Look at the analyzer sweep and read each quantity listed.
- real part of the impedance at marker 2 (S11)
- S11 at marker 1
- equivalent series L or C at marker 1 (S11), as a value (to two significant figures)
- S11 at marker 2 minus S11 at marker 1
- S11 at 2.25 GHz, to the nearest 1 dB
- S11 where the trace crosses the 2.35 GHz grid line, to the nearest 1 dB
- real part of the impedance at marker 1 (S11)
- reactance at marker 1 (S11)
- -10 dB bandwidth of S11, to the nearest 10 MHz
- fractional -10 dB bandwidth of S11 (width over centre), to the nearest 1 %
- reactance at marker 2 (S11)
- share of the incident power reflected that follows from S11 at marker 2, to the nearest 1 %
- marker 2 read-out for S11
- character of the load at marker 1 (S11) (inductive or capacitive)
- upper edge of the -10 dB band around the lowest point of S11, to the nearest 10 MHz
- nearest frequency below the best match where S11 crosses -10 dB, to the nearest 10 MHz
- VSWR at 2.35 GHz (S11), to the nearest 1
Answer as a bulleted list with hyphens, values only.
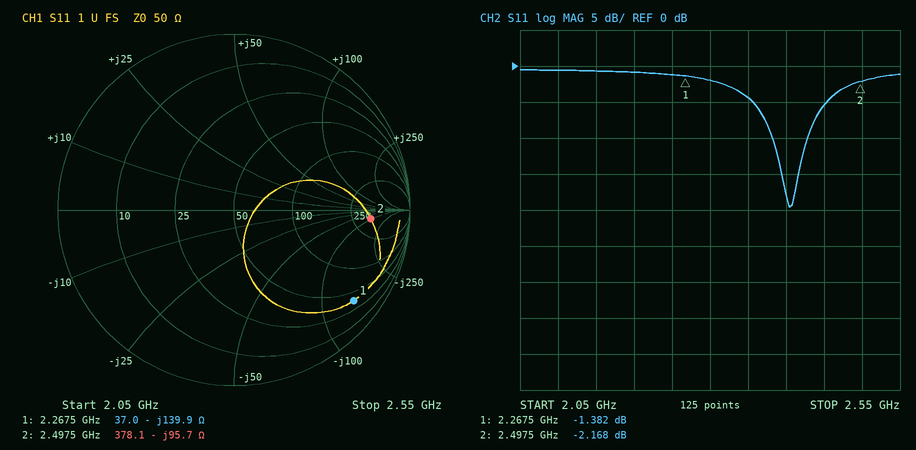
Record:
- 378.1 Ω
- -1.382 dB
- 500 fF
- -0.786 dB
- -1 dB
- -4 dB
- 37.0 Ω
- -139.9 Ω
- 50 MHz
- 2 %
- -95.7 Ω
- 61 %
- -2.168 dB
- capacitive
- 2.43 GHz
- 2.38 GHz
- 4
